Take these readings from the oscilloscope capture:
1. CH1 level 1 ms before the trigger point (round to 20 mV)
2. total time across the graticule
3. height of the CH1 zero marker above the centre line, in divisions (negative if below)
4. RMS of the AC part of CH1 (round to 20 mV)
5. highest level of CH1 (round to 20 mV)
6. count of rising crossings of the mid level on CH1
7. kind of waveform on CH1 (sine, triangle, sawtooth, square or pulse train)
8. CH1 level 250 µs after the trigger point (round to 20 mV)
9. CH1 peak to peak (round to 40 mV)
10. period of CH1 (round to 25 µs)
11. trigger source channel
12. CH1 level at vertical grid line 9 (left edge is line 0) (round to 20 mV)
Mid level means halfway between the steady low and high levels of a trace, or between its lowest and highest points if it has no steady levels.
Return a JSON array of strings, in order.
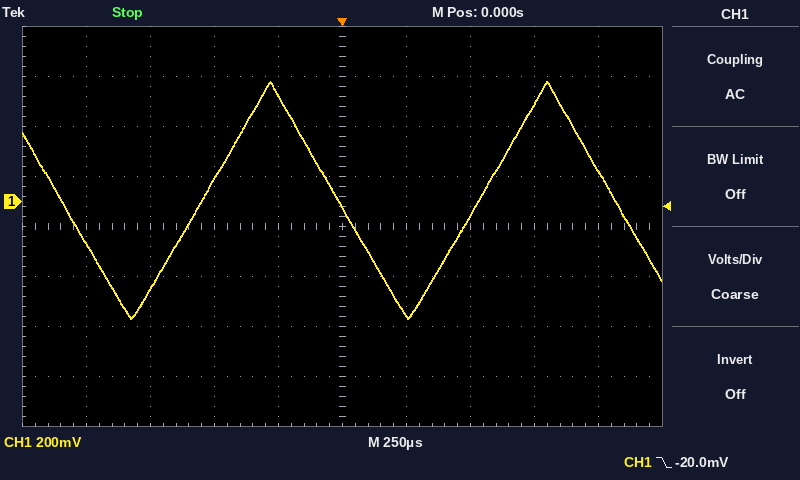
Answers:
["-160 mV", "2.5 ms", "+0.5 div", "280 mV", "480 mV", "2", "triangle", "-460 mV", "960 mV", "1.075 ms", "CH1", "120 mV"]
